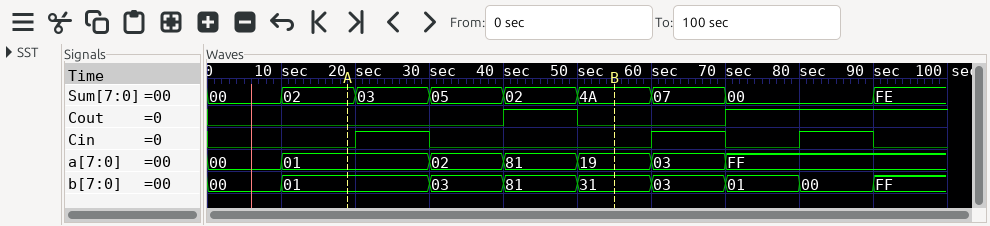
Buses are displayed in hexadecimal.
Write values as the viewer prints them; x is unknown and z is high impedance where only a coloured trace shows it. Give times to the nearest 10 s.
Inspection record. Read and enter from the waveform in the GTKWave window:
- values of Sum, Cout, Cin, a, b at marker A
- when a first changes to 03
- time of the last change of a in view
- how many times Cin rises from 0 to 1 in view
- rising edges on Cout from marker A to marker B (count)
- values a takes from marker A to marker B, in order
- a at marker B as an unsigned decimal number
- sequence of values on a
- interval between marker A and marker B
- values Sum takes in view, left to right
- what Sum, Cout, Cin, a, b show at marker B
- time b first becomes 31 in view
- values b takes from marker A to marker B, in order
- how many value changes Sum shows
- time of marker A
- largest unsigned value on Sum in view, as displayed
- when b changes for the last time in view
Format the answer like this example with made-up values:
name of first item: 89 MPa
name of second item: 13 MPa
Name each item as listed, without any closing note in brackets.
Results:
values of Sum, Cout, Cin, a, b at marker A: Sum=02, Cout=0, Cin=0, a=01, b=01
when a first changes to 03: 60 s
time of the last change of a in view: 70 s
how many times Cin rises from 0 to 1 in view: 3
rising edges on Cout from marker A to marker B: 1
values a takes from marker A to marker B, in order: 01, 02, 81, 19
a at marker B as an unsigned decimal number: 25
sequence of values on a: 00, 01, 02, 81, 19, 03, FF
interval between marker A and marker B: 40 s
values Sum takes in view, left to right: 00, 02, 03, 05, 02, 4A, 07, 00, FE
what Sum, Cout, Cin, a, b show at marker B: Sum=4A, Cout=0, Cin=0, a=19, b=31
time b first becomes 31 in view: 50 s
values b takes from marker A to marker B, in order: 01, 03, 81, 31
how many value changes Sum shows: 8
time of marker A: 20 s
largest unsigned value on Sum in view, as displayed: FE
when b changes for the last time in view: 90 s
